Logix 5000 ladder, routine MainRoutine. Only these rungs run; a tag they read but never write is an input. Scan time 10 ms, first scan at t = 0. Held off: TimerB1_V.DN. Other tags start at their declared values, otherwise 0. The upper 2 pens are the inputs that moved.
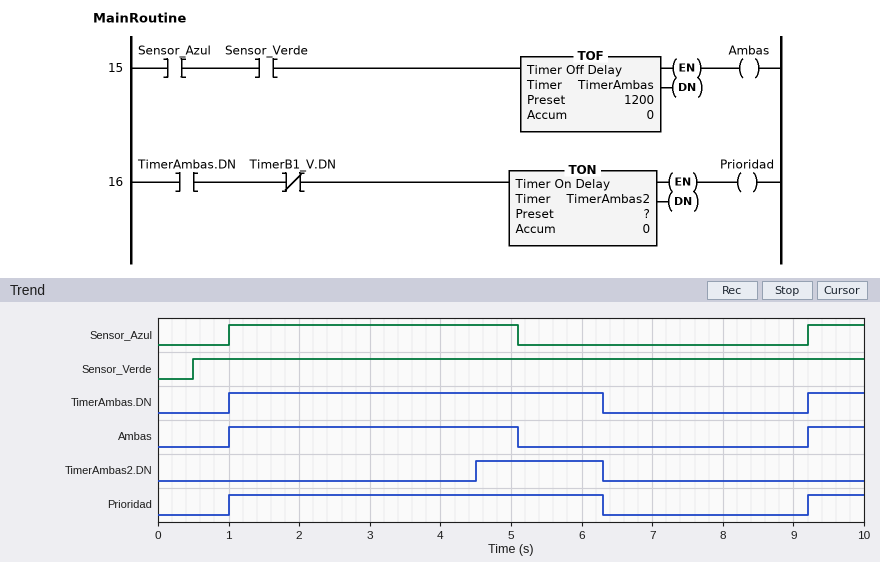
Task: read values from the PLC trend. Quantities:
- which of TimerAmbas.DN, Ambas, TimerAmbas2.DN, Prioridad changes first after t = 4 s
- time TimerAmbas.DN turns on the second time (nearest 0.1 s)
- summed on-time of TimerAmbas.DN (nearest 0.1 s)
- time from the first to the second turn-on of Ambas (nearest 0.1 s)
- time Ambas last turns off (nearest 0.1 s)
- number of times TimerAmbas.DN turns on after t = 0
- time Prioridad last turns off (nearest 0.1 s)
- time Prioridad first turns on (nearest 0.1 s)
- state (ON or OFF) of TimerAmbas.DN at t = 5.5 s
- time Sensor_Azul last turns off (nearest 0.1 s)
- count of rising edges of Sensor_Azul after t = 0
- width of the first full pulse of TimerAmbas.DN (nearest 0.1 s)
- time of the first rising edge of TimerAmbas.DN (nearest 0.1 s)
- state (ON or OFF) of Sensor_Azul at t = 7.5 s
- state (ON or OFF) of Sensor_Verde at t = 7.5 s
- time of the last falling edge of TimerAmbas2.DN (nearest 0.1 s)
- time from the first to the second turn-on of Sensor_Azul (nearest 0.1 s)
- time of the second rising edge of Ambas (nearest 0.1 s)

TimerAmbas2.DN
9.2 s
6.1 s
8.2 s
5.1 s
2
6.3 s
1.0 s
ON
5.1 s
2
5.3 s
1.0 s
OFF
ON
6.3 s
8.2 s
9.2 s
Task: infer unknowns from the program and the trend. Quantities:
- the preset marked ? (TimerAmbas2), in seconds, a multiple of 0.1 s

3.5 s
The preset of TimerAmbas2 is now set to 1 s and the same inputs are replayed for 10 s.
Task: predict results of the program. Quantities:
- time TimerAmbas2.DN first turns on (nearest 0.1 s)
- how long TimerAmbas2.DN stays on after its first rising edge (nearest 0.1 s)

2.0 s
4.3 s
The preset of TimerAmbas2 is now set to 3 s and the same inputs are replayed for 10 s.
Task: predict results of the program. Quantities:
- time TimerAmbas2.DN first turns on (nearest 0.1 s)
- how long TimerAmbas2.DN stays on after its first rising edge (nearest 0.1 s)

4.0 s
2.3 s
